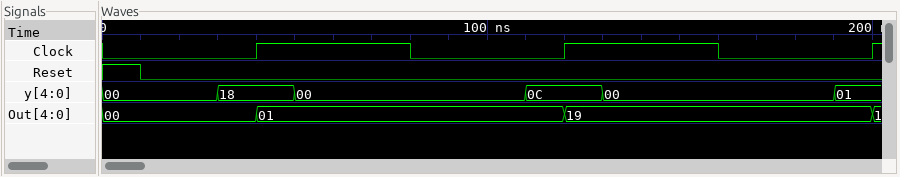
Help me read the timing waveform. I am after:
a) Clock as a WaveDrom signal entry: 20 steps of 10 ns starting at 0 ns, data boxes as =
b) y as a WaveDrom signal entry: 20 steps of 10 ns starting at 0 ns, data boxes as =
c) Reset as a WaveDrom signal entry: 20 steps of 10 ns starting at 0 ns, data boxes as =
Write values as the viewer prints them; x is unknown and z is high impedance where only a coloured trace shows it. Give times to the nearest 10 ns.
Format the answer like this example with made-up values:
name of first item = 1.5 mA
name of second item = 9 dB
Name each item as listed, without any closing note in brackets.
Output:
Clock as a WaveDrom signal entry: 20 steps of 10 ns starting at 0 ns, data boxes as = = {name: 'Clock', wave: '0...1...0...1...0...'}
y as a WaveDrom signal entry: 20 steps of 10 ns starting at 0 ns, data boxes as = = {name: 'y', wave: '=..=.=.....=.=.....=', data: '00 18 00 0C 00 01'}
Reset as a WaveDrom signal entry: 20 steps of 10 ns starting at 0 ns, data boxes as = = {name: 'Reset', wave: '10..................'}
